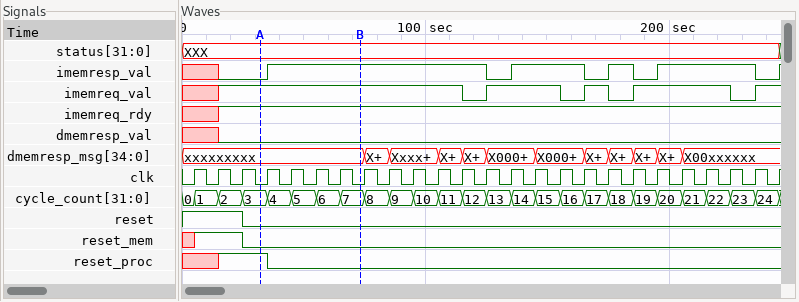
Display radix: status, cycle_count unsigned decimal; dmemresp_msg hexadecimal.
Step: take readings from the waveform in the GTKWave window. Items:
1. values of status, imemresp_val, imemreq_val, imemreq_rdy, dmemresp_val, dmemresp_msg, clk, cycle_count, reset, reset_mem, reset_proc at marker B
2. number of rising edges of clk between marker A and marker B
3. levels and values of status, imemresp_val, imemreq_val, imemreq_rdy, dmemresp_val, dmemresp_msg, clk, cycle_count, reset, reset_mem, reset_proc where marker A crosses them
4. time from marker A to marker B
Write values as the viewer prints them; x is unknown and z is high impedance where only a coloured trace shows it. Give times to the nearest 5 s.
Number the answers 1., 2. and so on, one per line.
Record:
1. status=XXX, imemresp_val=1, imemreq_val=1, imemreq_rdy=1, dmemresp_val=0, dmemresp_msg=xxxxxxxxx, clk=0, cycle_count=7, reset=0, reset_mem=0, reset_proc=0
2. 4
3. status=XXX, imemresp_val=0, imemreq_val=1, imemreq_rdy=1, dmemresp_val=0, dmemresp_msg=xxxxxxxxx, clk=0, cycle_count=3, reset=0, reset_mem=0, reset_proc=1
4. 40 s
